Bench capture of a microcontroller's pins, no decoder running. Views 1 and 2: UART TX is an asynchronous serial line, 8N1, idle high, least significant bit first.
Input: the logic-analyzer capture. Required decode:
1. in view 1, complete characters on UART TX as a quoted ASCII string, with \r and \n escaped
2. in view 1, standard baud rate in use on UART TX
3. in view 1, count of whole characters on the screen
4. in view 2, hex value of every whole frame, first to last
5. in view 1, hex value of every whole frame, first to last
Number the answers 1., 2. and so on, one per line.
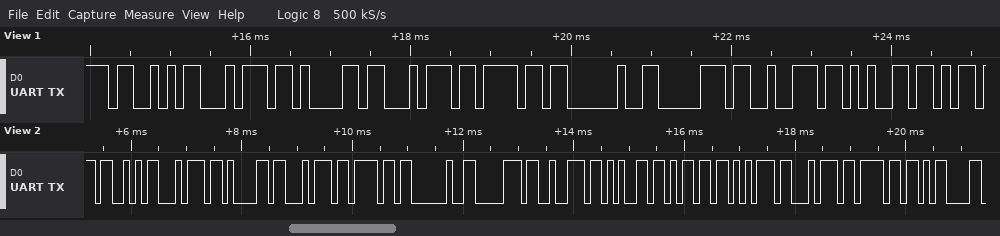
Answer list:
1. "Stato pre"
2. 9600 baud
3. 9
4. 53 74 61 74 6F 20 70 72 65 6D 75 74 6F 0D
5. 53 74 61 74 6F 20 70 72 65
